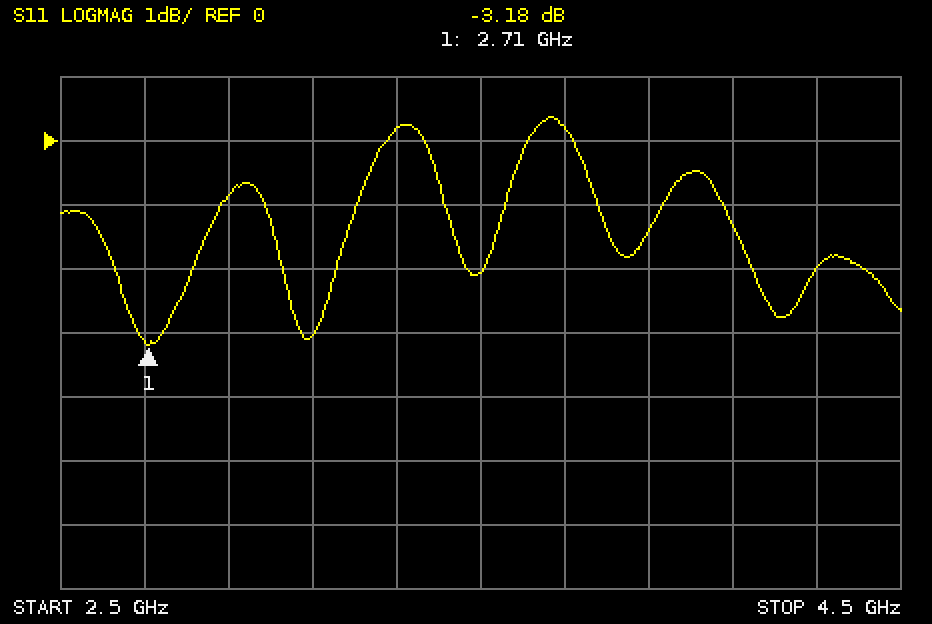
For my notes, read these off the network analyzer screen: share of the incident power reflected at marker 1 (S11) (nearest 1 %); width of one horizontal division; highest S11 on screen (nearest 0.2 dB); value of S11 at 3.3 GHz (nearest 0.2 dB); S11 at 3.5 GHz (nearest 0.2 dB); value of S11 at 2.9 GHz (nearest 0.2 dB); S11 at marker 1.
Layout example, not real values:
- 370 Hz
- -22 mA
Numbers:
- 48 %
- 200 MHz
- 0.4 dB
- 0.2 dB
- -2.0 dB
- -0.8 dB
- -3.18 dB
